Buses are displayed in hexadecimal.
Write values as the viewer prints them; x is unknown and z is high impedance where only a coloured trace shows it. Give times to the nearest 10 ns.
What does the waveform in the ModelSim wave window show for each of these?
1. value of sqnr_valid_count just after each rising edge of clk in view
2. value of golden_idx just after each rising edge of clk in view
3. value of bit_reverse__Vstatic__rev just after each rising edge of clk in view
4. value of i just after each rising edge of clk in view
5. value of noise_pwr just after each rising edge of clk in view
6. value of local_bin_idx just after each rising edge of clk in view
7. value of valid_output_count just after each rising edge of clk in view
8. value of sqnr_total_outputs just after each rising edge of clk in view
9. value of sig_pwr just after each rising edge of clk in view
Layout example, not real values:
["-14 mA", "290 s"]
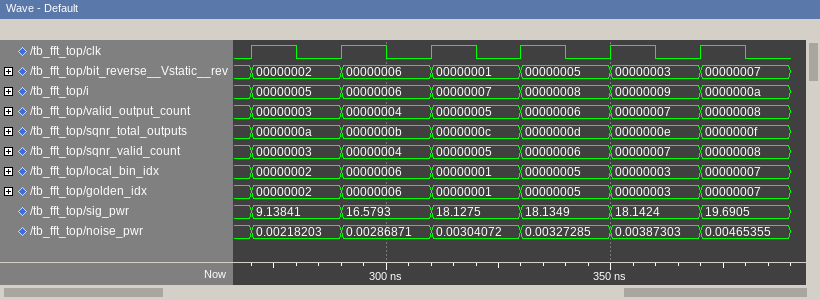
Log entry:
["00000003, 00000004, 00000005, 00000006, 00000007, 00000008", "00000002, 00000006, 00000001, 00000005, 00000003, 00000007", "00000002, 00000006, 00000001, 00000005, 00000003, 00000007", "00000005, 00000006, 00000007, 00000008, 00000009, 0000000a", "0.00218203, 0.00286871, 0.00304072, 0.00327285, 0.00387303, 0.00465355", "00000002, 00000006, 00000001, 00000005, 00000003, 00000007", "00000003, 00000004, 00000005, 00000006, 00000007, 00000008", "0000000a, 0000000b, 0000000c, 0000000d, 0000000e, 0000000f", "9.13841, 16.5793, 18.1275, 18.1349, 18.1424, 19.6905"]
